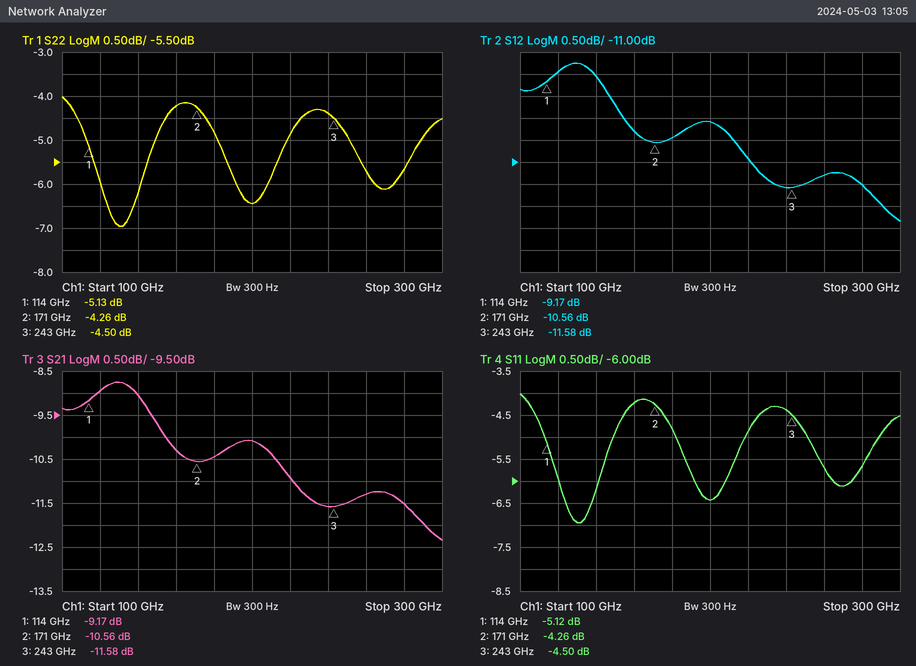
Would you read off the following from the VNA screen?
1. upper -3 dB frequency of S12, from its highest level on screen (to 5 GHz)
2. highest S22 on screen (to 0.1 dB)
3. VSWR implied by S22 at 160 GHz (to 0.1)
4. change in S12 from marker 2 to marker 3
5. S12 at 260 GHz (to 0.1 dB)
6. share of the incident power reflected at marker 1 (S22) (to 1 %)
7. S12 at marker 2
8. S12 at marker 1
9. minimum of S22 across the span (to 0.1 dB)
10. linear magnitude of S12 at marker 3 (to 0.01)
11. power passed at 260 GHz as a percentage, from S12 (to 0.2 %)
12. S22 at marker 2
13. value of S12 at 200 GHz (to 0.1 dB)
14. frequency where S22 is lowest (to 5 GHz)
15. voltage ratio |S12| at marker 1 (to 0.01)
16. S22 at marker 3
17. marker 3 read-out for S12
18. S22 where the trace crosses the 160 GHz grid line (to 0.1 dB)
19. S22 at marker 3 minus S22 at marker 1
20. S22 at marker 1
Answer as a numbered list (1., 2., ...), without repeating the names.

1. 285 GHz
2. -4.0 dB
3. 4.2
4. -1.02 dB
5. -11.3 dB
6. 31 %
7. -10.56 dB
8. -9.17 dB
9. -7.0 dB
10. 0.26
11. 7.4 %
12. -4.26 dB
13. -10.1 dB
14. 130 GHz
15. 0.35
16. -4.50 dB
17. -11.58 dB
18. -4.2 dB
19. 0.63 dB
20. -5.13 dB
